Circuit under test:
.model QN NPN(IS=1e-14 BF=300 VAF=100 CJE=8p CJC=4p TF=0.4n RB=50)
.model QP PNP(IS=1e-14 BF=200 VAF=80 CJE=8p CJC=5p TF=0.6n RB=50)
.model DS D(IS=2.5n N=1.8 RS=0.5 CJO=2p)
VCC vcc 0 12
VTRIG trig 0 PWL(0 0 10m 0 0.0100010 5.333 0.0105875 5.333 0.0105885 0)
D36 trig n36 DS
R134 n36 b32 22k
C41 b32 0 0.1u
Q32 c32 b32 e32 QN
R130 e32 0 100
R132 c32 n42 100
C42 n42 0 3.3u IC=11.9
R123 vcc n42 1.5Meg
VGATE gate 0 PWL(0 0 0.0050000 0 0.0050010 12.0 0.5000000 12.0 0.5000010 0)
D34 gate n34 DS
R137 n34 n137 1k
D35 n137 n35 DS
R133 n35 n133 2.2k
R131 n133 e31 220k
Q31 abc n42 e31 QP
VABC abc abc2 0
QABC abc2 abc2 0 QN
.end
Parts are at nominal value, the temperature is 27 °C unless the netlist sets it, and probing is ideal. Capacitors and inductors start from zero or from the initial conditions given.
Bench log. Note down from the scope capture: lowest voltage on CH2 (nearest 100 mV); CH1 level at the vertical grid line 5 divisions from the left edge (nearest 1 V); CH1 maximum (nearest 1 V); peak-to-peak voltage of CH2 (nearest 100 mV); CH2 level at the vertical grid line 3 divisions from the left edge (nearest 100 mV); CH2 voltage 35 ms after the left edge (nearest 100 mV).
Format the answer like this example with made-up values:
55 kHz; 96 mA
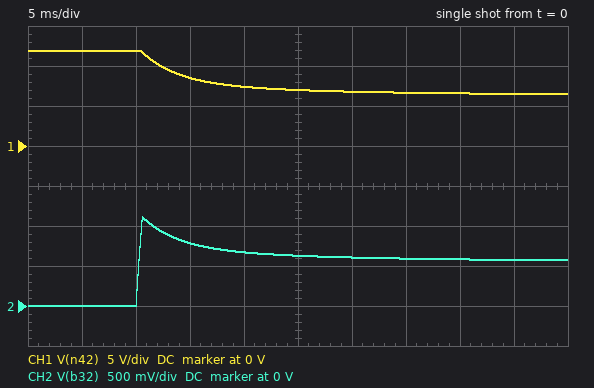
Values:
0 V; 7 V; 12 V; 1.1 V; 800 mV; 600 mV
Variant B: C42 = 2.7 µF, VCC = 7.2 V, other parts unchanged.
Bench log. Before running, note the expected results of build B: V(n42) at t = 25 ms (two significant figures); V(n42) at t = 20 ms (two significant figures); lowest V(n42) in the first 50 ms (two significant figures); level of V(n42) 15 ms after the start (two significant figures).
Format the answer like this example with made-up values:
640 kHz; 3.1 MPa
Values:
5.9 V; 6.4 V; 5.2 V; 7.7 V
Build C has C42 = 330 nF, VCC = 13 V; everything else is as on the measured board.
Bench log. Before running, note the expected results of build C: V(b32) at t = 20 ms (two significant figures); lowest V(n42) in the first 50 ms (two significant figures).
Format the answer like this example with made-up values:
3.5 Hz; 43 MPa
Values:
520 mV; 41 mV
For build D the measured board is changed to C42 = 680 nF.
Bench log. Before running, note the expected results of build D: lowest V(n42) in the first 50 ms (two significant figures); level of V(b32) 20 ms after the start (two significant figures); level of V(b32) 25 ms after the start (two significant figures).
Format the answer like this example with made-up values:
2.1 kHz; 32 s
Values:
50 mV; 520 mV; 510 mV
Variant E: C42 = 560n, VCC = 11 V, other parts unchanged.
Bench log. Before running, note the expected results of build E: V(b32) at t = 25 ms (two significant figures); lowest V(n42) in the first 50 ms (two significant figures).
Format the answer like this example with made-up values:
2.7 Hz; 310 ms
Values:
510 mV; 47 mV
